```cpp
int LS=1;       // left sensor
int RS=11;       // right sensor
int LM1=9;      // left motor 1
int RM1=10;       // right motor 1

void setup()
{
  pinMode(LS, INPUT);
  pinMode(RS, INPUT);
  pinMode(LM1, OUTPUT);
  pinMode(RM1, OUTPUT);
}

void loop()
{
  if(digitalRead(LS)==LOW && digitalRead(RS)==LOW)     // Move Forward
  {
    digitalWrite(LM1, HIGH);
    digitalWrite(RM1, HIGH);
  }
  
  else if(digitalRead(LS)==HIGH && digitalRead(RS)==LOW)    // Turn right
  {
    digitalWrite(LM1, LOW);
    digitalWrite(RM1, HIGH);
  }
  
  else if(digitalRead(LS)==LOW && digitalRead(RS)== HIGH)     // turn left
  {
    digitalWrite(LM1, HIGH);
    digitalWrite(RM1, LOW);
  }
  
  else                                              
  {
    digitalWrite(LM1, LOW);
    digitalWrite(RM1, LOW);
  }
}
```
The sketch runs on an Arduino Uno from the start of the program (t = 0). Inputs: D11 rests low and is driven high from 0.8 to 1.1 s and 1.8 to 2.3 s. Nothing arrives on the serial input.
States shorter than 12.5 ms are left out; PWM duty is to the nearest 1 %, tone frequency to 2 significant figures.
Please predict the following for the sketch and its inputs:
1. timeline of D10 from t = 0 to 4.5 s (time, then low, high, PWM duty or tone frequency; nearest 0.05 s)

0 s high; 0.8 s low; 1.1 s high; 1.8 s low; 2.3 s high
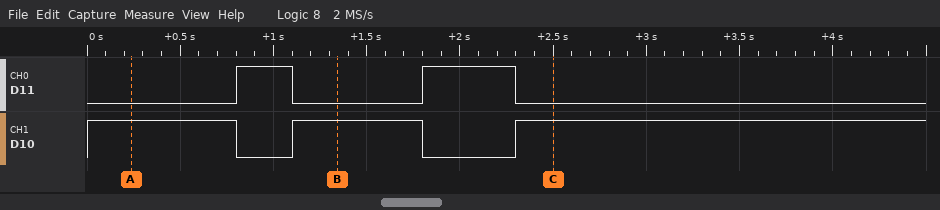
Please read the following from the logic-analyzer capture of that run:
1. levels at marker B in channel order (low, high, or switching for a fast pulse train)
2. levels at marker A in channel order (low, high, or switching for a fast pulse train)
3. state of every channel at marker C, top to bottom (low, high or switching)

D11 low, D10 high
D11 low, D10 high
D11 low, D10 high
